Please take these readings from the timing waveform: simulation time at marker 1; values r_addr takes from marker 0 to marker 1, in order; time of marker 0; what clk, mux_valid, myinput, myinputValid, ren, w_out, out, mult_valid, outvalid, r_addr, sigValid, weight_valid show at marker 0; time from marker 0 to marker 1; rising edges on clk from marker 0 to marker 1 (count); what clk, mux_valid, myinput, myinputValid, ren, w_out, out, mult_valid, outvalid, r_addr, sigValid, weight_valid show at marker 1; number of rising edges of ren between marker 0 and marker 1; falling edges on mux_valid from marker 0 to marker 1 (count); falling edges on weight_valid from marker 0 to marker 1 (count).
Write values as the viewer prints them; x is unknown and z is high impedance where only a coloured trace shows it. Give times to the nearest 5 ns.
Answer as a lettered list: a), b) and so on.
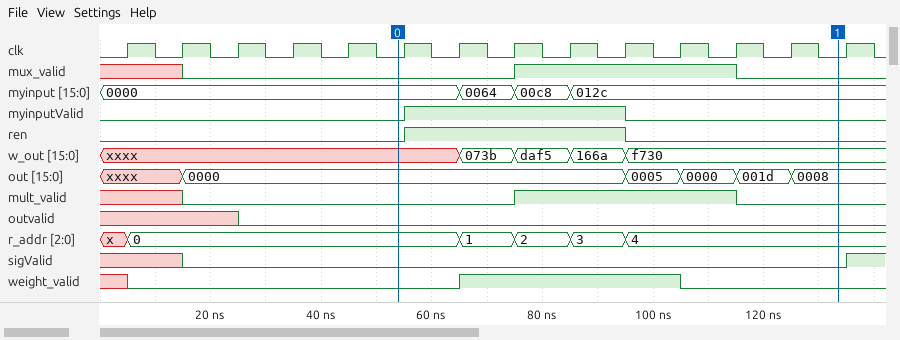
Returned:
a) 135 ns
b) 0, 1, 2, 3, 4
c) 55 ns
d) clk=0, mux_valid=0, myinput=0000, myinputValid=0, ren=0, w_out=xxxx, out=0000, mult_valid=0, outvalid=0, r_addr=0, sigValid=0, weight_valid=0
e) 80 ns
f) 8
g) clk=0, mux_valid=0, myinput=012c, myinputValid=0, ren=0, w_out=f730, out=0008, mult_valid=0, outvalid=0, r_addr=4, sigValid=0, weight_valid=0
h) 1
i) 1
j) 1
